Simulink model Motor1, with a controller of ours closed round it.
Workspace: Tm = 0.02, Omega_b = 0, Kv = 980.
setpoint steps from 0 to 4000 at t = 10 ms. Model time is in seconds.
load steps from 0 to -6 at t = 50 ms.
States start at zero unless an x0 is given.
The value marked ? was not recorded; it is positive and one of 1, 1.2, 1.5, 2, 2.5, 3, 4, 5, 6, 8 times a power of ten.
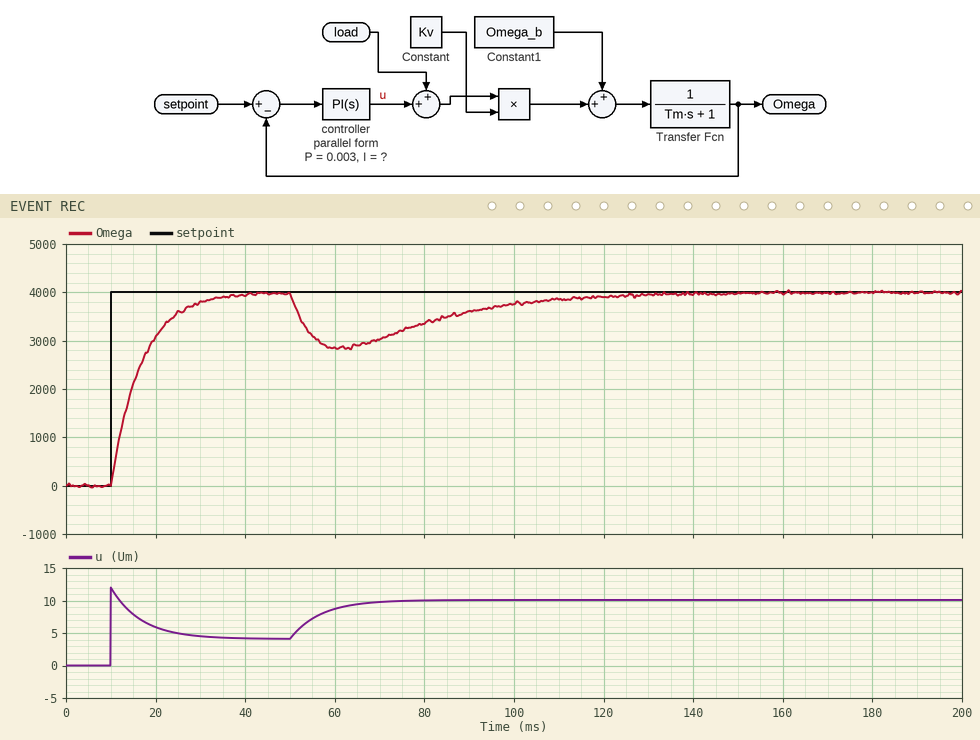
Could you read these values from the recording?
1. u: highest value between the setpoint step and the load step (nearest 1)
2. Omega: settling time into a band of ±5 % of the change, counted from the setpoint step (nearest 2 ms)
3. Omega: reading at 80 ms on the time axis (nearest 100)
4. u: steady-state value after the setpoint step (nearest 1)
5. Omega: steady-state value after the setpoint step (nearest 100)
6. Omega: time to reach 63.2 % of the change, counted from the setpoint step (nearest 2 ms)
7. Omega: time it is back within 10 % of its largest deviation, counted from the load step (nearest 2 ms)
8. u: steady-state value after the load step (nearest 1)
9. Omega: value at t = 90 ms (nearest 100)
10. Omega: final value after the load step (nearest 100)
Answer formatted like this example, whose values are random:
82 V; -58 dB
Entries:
12; 20 ms; 3400; 4; 4000; 6 ms; 66 ms; 10; 3600; 4000
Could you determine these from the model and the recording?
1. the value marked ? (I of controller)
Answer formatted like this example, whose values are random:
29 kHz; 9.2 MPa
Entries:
0.15
